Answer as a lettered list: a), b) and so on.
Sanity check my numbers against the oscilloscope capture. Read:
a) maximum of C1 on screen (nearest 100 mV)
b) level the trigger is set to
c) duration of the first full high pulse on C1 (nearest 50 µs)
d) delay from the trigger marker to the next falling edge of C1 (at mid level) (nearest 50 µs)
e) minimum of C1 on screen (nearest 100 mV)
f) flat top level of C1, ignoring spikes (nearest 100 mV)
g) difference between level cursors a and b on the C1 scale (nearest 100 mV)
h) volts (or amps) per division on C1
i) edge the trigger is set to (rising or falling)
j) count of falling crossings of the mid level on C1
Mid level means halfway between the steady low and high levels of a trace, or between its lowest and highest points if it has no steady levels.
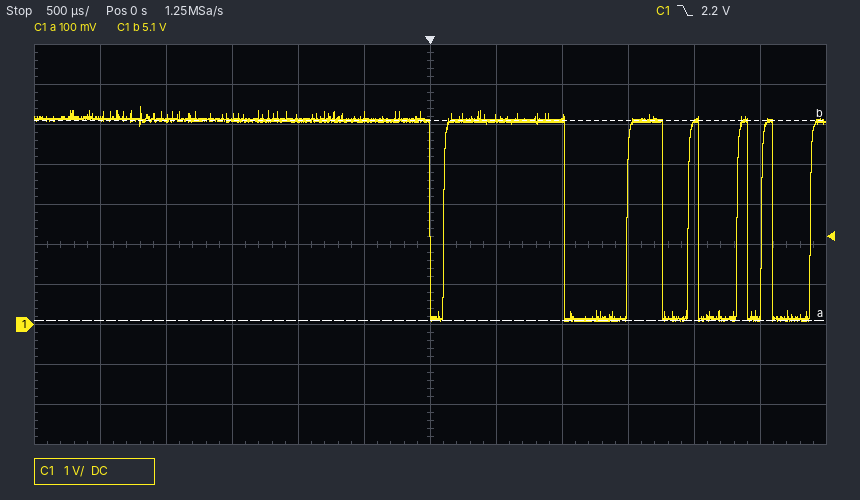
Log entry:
a) 5.4 V
b) 2.2 V
c) 900 µs
d) 1.00 ms
e) 100 mV
f) 5.1 V
g) 5.0 V
h) 1 V
i) falling
j) 6
